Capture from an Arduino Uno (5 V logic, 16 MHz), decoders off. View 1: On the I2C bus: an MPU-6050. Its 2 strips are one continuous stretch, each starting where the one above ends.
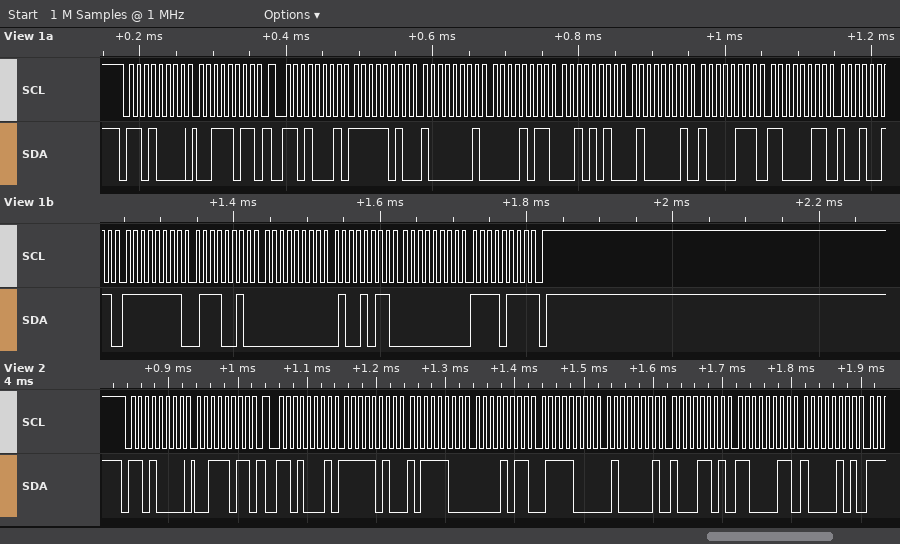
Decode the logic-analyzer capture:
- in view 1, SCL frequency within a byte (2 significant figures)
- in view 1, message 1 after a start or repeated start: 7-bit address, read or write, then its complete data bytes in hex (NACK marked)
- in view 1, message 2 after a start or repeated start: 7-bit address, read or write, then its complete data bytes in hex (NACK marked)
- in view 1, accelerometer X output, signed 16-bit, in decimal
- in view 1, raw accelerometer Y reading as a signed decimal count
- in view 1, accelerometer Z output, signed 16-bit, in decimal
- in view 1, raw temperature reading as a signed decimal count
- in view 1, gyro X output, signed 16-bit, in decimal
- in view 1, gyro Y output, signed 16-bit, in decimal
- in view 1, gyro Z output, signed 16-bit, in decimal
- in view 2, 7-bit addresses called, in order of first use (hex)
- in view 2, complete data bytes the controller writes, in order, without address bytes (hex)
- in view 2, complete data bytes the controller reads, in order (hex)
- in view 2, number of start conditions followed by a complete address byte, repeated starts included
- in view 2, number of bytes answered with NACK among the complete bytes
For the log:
100 kHz
0x68 write: 3B
0x68 read: FA 81 0B 2A 41 87 C3 93 FF 72 00 4B 00 F7 NACK
-1407
2858
16775
-15469
-142
75
247
0x68
3B
FA BC 0B 78 41 8D C3 85
2
0
